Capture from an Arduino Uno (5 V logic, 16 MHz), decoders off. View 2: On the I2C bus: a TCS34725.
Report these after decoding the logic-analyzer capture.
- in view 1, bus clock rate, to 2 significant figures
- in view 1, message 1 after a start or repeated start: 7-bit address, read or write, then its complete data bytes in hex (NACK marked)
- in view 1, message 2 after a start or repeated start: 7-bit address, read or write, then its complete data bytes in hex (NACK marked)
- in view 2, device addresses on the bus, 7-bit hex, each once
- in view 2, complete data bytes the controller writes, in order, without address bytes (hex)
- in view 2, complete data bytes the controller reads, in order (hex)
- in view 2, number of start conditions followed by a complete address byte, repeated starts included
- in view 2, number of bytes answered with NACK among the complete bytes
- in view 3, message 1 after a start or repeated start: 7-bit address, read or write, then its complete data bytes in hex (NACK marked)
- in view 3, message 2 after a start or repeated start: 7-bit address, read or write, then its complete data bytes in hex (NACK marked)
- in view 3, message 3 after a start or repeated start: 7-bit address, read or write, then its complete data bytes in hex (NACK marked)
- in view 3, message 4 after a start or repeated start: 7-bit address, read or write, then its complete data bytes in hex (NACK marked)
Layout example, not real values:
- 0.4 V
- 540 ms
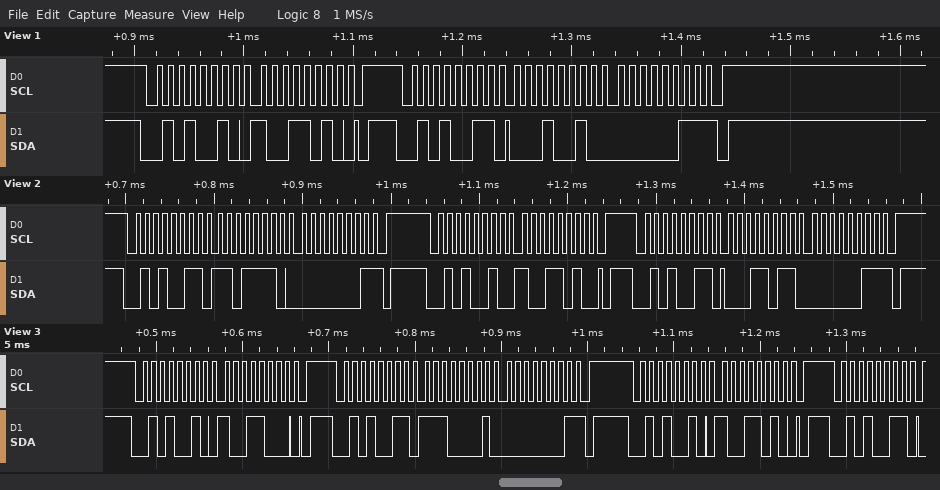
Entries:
- 100 kHz
- 0x29 write: 9A
- 0x29 read: 12 03 NACK
- 0x29
- 9A
- DE 01 1B 03
- 3
- 2
- 0x29 write: 98
- 0x29 read: E1 01 NACK
- 0x29 write: 9A
- 0x29 read
